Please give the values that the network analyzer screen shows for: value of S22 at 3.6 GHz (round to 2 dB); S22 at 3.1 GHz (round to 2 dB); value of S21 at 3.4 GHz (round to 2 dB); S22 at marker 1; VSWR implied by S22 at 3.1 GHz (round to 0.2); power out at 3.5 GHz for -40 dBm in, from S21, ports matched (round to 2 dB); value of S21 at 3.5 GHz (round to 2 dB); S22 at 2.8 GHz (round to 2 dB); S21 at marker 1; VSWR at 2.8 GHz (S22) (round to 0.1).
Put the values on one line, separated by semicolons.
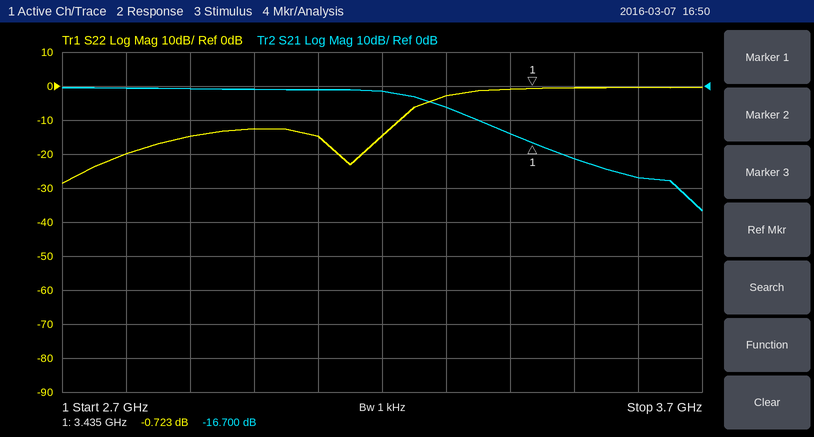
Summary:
0 dB; -14 dB; -14 dB; -0.723 dB; 1.4; -62 dBm; -22 dB; -20 dB; -16.700 dB; 1.2
